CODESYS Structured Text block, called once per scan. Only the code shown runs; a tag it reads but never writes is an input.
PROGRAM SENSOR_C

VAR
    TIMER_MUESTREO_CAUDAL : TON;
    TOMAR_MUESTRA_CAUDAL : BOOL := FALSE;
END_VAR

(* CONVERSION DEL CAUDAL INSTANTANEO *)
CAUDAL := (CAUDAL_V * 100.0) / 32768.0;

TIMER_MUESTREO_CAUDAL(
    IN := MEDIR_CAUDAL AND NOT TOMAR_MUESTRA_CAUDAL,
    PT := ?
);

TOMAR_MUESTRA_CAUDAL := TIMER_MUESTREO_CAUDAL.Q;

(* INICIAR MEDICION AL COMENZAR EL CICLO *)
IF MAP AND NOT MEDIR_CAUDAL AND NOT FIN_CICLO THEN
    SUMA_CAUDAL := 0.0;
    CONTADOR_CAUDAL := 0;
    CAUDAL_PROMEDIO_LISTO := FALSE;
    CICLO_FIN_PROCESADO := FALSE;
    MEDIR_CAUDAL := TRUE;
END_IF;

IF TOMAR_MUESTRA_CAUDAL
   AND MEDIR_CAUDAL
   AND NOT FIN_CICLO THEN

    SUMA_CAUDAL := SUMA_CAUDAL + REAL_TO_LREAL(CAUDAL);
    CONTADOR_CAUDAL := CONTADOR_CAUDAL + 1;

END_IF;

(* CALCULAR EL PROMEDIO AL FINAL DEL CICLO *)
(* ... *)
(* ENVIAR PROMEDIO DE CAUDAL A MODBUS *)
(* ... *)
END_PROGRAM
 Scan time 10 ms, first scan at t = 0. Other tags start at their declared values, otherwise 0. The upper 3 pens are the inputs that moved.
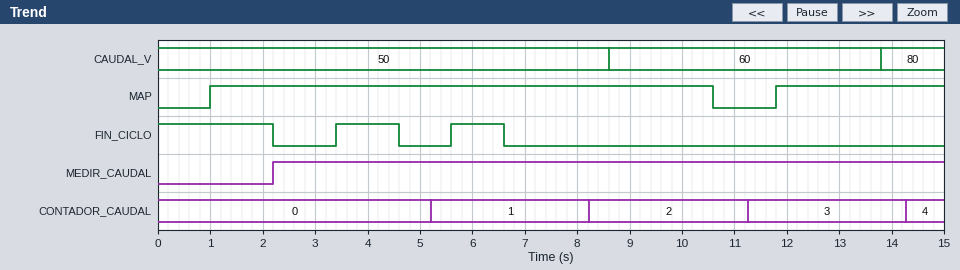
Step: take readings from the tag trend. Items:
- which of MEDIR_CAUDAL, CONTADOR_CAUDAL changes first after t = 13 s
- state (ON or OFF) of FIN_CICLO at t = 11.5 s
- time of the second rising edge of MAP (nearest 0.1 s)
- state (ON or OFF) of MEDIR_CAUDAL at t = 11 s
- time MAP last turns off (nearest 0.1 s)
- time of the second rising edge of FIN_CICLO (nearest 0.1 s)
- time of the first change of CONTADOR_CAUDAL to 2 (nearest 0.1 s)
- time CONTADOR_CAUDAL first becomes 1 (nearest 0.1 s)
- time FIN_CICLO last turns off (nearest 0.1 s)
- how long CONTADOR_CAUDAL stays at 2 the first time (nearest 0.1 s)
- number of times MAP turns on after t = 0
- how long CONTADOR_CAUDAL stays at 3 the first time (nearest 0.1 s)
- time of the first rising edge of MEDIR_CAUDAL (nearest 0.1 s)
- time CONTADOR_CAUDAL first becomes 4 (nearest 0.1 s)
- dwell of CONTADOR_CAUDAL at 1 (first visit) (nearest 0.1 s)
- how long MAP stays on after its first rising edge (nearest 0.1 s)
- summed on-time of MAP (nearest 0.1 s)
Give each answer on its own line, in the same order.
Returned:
CONTADOR_CAUDAL
OFF
11.8 s
ON
10.6 s
5.6 s
8.2 s
5.2 s
6.6 s
3.0 s
2
3.0 s
2.2 s
14.3 s
3.0 s
9.6 s
12.8 s
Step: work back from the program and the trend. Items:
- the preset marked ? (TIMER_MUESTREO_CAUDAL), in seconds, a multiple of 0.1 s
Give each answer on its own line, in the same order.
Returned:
3.0 s
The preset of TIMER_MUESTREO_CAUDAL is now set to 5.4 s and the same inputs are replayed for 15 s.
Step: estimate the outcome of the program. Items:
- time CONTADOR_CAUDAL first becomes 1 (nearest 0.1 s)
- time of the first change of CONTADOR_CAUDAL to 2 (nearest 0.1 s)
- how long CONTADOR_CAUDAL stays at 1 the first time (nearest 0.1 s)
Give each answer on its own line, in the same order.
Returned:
7.6 s
13.0 s
5.4 s
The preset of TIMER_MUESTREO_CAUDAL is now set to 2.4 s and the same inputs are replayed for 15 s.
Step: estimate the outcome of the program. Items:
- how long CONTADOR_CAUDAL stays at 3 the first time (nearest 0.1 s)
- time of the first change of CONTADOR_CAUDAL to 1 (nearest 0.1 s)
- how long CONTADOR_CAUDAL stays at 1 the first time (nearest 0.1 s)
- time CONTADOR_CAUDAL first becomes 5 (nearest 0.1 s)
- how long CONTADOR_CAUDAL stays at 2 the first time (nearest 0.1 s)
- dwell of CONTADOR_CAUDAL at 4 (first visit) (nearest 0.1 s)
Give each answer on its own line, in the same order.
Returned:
2.4 s
4.6 s
2.4 s
14.3 s
2.4 s
2.4 s
